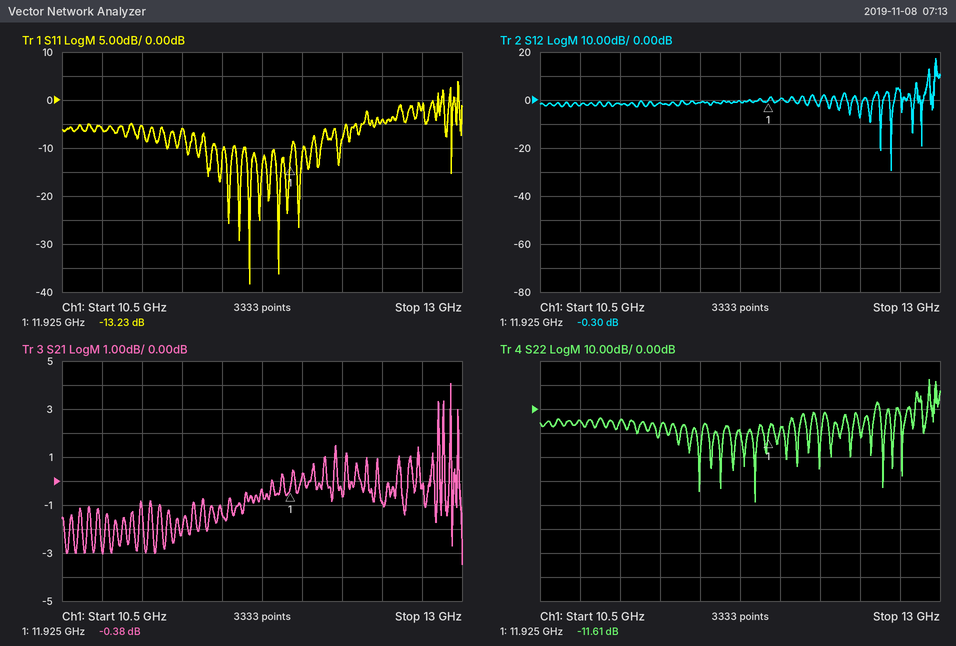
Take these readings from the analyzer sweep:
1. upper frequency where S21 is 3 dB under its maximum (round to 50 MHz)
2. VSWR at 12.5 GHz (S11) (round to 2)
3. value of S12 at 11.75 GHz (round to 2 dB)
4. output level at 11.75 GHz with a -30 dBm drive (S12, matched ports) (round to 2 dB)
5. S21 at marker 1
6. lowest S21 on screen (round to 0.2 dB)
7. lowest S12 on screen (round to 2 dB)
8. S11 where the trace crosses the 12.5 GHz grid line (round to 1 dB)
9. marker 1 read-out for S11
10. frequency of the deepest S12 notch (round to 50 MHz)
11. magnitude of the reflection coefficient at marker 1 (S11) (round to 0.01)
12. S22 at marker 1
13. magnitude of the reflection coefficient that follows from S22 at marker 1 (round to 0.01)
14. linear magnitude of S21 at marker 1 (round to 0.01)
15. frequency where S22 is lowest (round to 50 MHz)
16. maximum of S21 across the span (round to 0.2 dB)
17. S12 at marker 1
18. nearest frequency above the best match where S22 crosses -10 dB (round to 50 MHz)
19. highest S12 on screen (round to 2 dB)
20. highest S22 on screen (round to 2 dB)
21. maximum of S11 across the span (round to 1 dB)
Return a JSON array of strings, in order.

["12.95 GHz", "4", "0 dB", "-30 dBm", "-0.38 dB", "-3.4 dB", "-30 dB", "-4 dB", "-13.23 dB", "12.70 GHz", "0.22", "-11.61 dB", "0.26", "0.96", "11.85 GHz", "4.0 dB", "-0.30 dB", "11.85 GHz", "18 dB", "12 dB", "4 dB"]
